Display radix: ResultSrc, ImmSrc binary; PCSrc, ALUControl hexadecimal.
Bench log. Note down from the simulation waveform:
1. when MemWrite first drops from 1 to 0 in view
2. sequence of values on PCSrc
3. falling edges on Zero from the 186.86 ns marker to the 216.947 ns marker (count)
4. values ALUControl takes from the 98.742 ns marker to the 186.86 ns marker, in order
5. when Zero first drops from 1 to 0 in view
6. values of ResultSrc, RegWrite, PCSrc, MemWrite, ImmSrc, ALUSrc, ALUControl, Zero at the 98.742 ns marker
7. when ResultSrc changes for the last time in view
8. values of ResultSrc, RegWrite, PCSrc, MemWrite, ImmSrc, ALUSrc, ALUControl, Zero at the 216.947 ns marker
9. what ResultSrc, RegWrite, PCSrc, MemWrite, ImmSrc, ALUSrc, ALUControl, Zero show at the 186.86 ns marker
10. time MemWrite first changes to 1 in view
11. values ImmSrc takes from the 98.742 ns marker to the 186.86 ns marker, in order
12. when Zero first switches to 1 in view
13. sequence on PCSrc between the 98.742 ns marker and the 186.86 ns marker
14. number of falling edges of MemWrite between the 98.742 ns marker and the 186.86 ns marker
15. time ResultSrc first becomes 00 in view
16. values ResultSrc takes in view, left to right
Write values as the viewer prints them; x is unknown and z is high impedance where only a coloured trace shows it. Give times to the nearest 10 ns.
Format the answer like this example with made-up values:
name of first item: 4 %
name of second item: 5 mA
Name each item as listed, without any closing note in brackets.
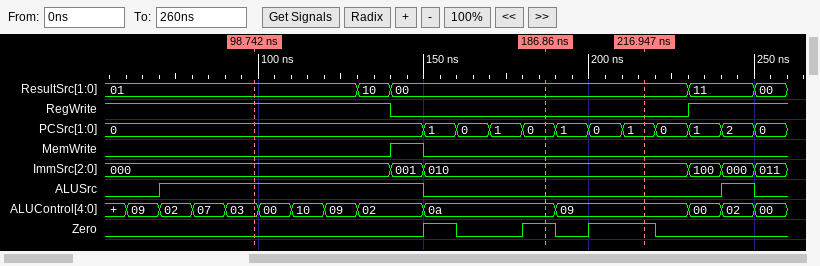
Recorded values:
when MemWrite first drops from 1 to 0 in view: 150 ns
sequence of values on PCSrc: 0, 1, 0, 1, 0, 1, 0, 1, 0, 1, 2, 0
falling edges on Zero from the 186.86 ns marker to the 216.947 ns marker: 1
values ALUControl takes from the 98.742 ns marker to the 186.86 ns marker, in order: 03, 00, 10, 09, 02, 0a
when Zero first drops from 1 to 0 in view: 160 ns
values of ResultSrc, RegWrite, PCSrc, MemWrite, ImmSrc, ALUSrc, ALUControl, Zero at the 98.742 ns marker: ResultSrc=01, RegWrite=1, PCSrc=0, MemWrite=0, ImmSrc=000, ALUSrc=1, ALUControl=03, Zero=0
when ResultSrc changes for the last time in view: 250 ns
values of ResultSrc, RegWrite, PCSrc, MemWrite, ImmSrc, ALUSrc, ALUControl, Zero at the 216.947 ns marker: ResultSrc=00, RegWrite=0, PCSrc=1, MemWrite=0, ImmSrc=010, ALUSrc=0, ALUControl=09, Zero=1
what ResultSrc, RegWrite, PCSrc, MemWrite, ImmSrc, ALUSrc, ALUControl, Zero show at the 186.86 ns marker: ResultSrc=00, RegWrite=0, PCSrc=0, MemWrite=0, ImmSrc=010, ALUSrc=0, ALUControl=0a, Zero=1
time MemWrite first changes to 1 in view: 140 ns
values ImmSrc takes from the 98.742 ns marker to the 186.86 ns marker, in order: 000, 001, 010
when Zero first switches to 1 in view: 150 ns
sequence on PCSrc between the 98.742 ns marker and the 186.86 ns marker: 0, 1, 0, 1, 0
number of falling edges of MemWrite between the 98.742 ns marker and the 186.86 ns marker: 1
time ResultSrc first becomes 00 in view: 140 ns
values ResultSrc takes in view, left to right: 01, 10, 00, 11, 00
